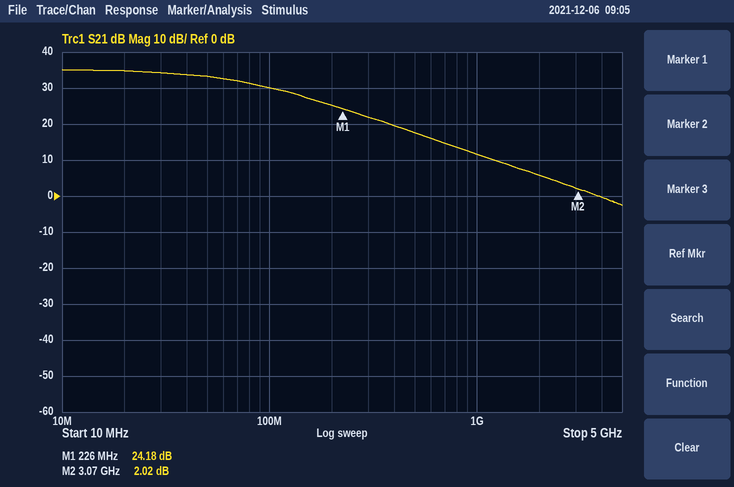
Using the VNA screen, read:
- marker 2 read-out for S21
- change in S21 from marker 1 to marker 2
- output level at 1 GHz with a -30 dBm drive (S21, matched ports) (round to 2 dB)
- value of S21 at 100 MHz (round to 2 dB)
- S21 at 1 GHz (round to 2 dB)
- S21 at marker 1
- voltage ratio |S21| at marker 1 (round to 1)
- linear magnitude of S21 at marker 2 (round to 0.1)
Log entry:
2.02 dB
-22.16 dB
-18 dBm
30 dB
12 dB
24.18 dB
16
1.3
